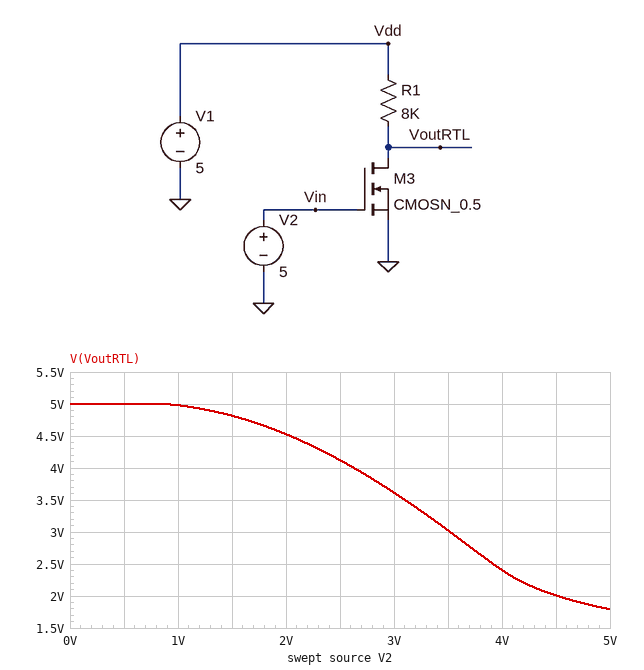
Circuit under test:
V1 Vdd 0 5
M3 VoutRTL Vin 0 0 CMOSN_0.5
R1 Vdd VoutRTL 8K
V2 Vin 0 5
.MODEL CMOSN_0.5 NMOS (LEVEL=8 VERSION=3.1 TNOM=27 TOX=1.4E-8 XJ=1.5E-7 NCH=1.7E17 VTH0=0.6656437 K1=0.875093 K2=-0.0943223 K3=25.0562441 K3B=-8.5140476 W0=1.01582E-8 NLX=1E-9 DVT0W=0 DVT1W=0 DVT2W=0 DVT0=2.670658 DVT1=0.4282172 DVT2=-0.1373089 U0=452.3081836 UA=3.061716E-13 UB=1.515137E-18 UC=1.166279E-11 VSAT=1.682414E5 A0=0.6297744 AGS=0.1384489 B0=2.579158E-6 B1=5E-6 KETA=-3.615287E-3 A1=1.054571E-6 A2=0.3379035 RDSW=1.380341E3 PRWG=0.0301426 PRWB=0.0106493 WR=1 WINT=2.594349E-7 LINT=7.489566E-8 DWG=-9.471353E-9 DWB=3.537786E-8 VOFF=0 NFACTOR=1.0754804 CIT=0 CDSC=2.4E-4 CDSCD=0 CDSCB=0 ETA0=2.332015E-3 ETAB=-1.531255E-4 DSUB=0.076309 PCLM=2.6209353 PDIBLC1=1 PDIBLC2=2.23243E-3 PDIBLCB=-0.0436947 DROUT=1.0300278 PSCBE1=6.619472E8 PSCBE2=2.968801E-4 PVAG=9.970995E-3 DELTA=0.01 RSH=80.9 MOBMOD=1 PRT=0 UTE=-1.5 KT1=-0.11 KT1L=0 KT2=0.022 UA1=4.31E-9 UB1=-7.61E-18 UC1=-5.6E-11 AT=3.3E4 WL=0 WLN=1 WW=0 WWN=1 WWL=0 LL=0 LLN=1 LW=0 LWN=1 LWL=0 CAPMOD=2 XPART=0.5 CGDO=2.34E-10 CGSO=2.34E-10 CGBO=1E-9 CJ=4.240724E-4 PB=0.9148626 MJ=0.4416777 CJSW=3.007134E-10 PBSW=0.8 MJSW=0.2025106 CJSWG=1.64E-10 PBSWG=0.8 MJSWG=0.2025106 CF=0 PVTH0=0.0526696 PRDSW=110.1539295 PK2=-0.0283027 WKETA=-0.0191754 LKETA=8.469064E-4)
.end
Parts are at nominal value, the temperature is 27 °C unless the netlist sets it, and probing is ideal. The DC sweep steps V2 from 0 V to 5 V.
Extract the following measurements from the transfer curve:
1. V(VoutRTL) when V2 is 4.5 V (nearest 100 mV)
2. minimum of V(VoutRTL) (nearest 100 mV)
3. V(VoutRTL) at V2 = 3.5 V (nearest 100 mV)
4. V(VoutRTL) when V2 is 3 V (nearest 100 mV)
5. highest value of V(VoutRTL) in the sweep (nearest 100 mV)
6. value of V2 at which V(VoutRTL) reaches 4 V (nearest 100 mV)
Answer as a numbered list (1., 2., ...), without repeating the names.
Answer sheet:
1. 2.0 V
2. 1.8 V
3. 3.0 V
4. 3.6 V
5. 5.0 V
6. 2.6 V
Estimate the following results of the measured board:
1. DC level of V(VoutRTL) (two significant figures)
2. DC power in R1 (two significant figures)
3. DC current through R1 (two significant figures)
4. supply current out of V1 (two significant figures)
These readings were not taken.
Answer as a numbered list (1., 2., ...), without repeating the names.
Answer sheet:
1. 1.8 V
2. 1.3 mW
3. 400 µA
4. 400 µA
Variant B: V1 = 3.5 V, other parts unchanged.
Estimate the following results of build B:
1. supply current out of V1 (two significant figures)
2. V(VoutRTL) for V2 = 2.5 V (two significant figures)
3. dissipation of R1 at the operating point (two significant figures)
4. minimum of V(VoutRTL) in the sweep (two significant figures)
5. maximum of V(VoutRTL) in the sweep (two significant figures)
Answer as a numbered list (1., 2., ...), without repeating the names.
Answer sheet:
1. 290 µA
2. 2.6 V
3. 680 µW
4. 1.2 V
5. 3.5 V
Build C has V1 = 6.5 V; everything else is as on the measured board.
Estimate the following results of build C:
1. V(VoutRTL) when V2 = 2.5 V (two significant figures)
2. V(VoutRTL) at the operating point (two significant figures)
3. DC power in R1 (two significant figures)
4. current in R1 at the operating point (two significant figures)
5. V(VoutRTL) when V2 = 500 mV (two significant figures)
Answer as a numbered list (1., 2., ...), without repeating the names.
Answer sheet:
1. 5.6 V
2. 2.6 V
3. 1.9 mW
4. 490 µA
5. 6.5 V
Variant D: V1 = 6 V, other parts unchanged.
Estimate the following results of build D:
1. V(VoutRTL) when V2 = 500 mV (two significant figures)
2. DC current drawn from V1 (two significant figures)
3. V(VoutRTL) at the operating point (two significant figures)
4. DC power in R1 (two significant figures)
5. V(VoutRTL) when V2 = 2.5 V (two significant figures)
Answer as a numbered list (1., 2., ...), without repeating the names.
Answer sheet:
1. 6.0 V
2. 460 µA
3. 2.3 V
4. 1.7 mW
5. 5.1 V
